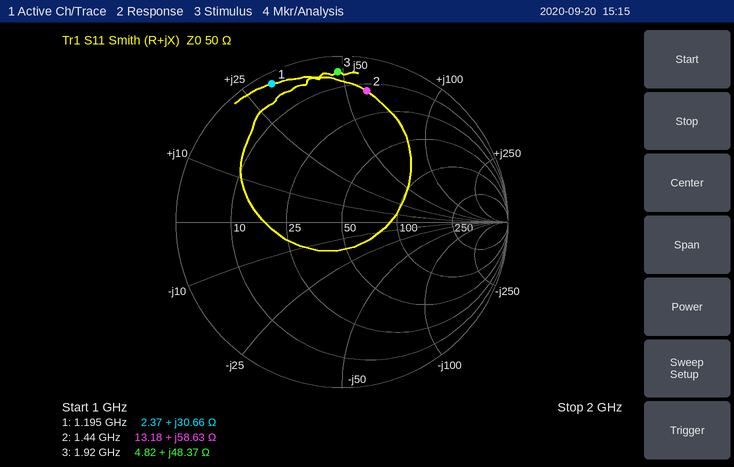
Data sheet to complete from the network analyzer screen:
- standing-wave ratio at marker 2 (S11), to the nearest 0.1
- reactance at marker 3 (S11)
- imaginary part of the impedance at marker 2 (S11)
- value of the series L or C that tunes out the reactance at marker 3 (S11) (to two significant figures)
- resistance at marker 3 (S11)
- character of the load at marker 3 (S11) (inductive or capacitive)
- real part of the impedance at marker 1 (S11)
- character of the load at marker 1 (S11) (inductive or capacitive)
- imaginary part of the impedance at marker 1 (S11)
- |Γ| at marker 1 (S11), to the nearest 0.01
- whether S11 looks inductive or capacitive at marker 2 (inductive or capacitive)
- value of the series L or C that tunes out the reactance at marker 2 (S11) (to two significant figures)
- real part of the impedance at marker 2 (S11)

9.2
+48.37 Ω
+58.63 Ω
1.7 pF
4.82 Ω
inductive
2.37 Ω
inductive
+30.66 Ω
0.93
inductive
1.9 pF
13.18 Ω
